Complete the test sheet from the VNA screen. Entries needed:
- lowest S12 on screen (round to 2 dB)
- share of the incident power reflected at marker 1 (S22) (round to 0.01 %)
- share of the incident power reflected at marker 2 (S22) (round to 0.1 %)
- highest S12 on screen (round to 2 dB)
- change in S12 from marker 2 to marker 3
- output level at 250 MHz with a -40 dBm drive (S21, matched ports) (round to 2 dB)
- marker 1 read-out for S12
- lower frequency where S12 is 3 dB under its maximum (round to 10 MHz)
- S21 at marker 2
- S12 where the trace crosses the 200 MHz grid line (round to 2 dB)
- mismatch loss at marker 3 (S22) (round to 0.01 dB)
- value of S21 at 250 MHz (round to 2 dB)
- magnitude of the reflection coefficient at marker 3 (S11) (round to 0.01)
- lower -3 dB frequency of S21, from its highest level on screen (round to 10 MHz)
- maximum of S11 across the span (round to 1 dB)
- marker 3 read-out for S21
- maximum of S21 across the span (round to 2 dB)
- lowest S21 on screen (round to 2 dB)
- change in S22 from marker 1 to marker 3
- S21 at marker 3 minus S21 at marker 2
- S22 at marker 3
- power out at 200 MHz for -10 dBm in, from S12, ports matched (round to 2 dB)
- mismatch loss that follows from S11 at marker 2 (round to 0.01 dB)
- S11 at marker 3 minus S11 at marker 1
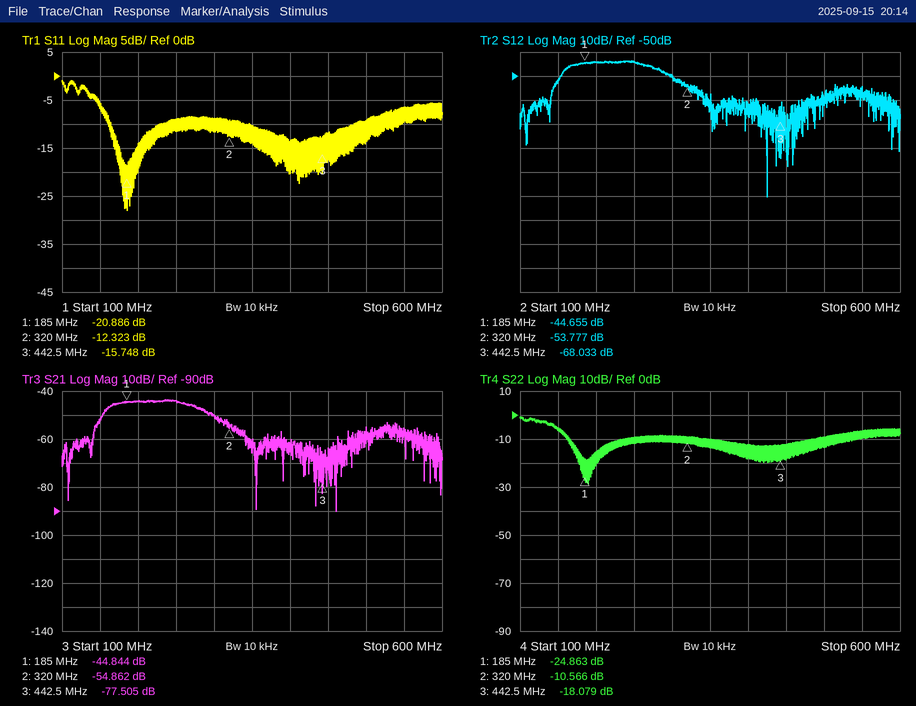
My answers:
-100 dB
0.33 %
8.8 %
-44 dB
-14.256 dB
-84 dBm
-44.655 dB
160 MHz
-54.862 dB
-44 dB
0.07 dB
-44 dB
0.16
160 MHz
-1 dB
-77.505 dB
-44 dB
-90 dB
6.784 dB
-22.643 dB
-18.079 dB
-54 dBm
0.26 dB
5.138 dB
